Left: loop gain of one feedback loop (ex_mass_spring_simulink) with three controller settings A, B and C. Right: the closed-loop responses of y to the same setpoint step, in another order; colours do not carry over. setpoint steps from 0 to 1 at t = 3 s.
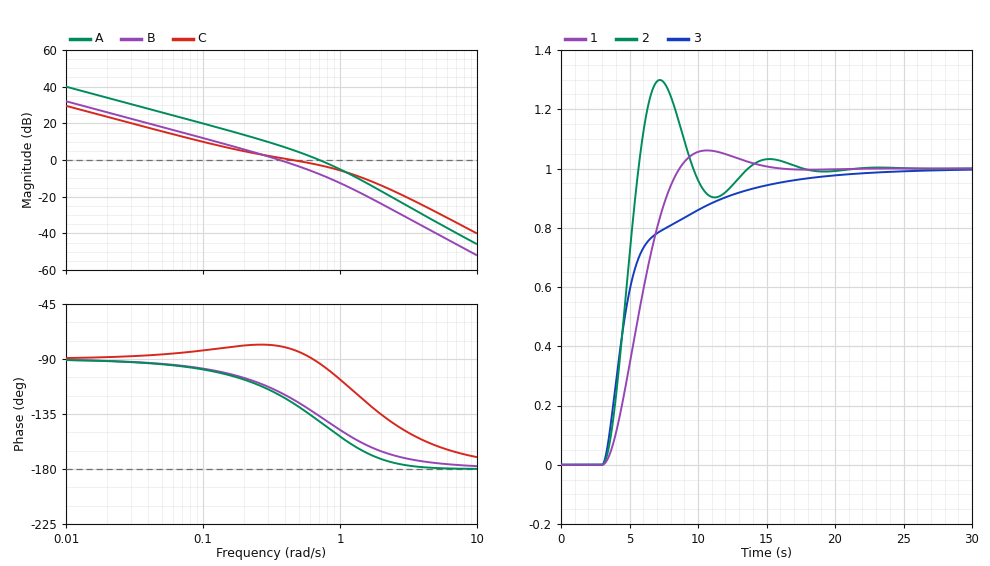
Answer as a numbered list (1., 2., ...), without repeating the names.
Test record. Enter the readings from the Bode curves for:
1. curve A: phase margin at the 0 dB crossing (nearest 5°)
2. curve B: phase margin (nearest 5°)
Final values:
1. 40°
2. 65°
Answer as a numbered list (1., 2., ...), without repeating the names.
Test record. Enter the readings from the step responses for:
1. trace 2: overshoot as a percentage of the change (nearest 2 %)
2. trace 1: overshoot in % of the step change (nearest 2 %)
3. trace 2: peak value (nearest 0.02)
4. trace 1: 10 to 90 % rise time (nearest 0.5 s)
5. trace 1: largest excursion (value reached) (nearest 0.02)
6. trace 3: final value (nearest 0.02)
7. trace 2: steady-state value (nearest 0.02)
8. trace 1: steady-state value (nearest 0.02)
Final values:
1. 30 %
2. 6 %
3. 1.30
4. 3.5 s
5. 1.06
6. 1.00
7. 1.00
8. 1.00
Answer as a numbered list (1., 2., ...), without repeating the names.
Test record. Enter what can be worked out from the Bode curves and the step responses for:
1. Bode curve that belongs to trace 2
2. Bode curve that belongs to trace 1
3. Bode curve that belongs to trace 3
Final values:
1. A
2. B
3. C
